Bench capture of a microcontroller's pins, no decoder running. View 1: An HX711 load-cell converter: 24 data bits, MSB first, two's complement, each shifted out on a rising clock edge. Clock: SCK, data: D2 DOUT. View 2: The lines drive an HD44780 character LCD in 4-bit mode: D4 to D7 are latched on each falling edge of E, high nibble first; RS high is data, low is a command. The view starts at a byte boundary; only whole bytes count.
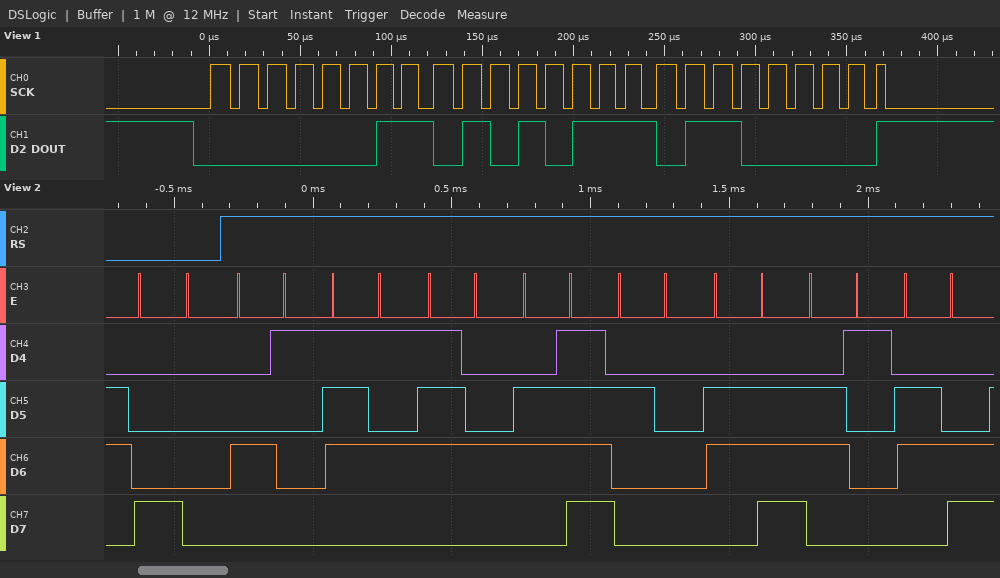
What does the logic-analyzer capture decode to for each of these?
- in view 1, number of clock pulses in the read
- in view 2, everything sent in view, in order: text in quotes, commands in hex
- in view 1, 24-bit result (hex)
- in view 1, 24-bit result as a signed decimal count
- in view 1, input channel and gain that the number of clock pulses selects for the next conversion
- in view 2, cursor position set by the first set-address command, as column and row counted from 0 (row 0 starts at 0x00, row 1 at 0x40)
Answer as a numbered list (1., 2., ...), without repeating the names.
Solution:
1. 25
2. 0x80 "Auto nal"
3. 0x035760
4. 218976
5. channel A, gain 128
6. column 0, row 0
